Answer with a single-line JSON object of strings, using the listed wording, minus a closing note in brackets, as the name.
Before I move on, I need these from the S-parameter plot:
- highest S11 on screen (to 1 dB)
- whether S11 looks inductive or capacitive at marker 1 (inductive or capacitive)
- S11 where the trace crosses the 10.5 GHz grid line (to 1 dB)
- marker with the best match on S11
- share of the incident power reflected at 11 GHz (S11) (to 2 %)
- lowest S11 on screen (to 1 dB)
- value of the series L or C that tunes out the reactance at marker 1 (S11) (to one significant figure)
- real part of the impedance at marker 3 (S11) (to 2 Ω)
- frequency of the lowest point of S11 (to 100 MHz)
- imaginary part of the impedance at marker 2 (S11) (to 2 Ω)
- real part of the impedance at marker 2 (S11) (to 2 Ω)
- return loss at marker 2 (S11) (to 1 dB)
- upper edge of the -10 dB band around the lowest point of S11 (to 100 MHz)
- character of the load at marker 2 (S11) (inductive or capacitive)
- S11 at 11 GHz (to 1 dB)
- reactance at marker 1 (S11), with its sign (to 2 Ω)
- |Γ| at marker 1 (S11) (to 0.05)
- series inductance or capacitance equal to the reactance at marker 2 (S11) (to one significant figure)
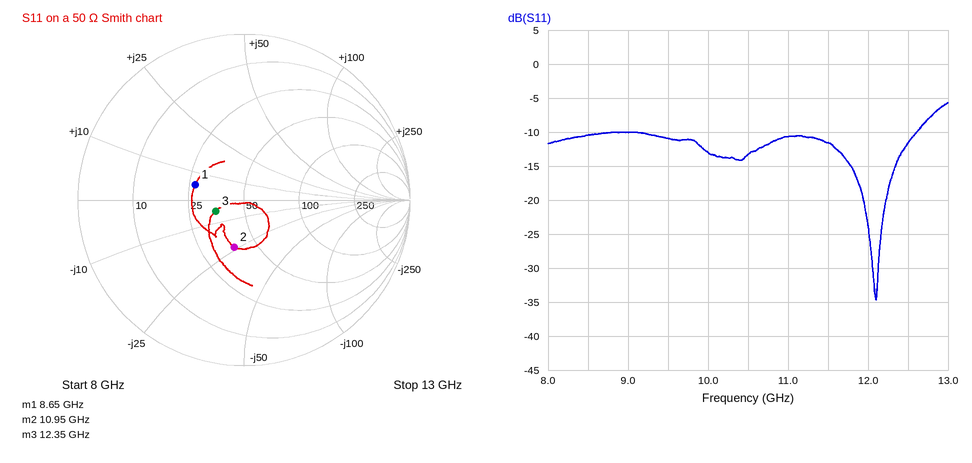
{"highest S11 on screen": "-6 dB", "whether S11 looks inductive or capacitive at marker 1": "inductive", "S11 where the trace crosses the 10.5 GHz grid line": "-13 dB", "marker with the best match on S11": "marker 3", "share of the incident power reflected at 11 GHz (S11)": "8 %", "lowest S11 on screen": "-35 dB", "value of the series L or C that tunes out the reactance at marker 1 (S11)": "3 pF", "real part of the impedance at marker 3 (S11)": "36 Ω", "frequency of the lowest point of S11": "12.1 GHz", "imaginary part of the impedance at marker 2 (S11)": "-24 Ω", "real part of the impedance at marker 2 (S11)": "38 Ω", "return loss at marker 2 (S11)": "11 dB", "upper edge of the -10 dB band around the lowest point of S11": "12.6 GHz", "character of the load at marker 2 (S11)": "capacitive", "S11 at 11 GHz": "-11 dB", "reactance at marker 1 (S11), with its sign": "+6 Ω", "|Γ| at marker 1 (S11)": "0.30", "series inductance or capacitance equal to the reactance at marker 2 (S11)": "600 fF"}
